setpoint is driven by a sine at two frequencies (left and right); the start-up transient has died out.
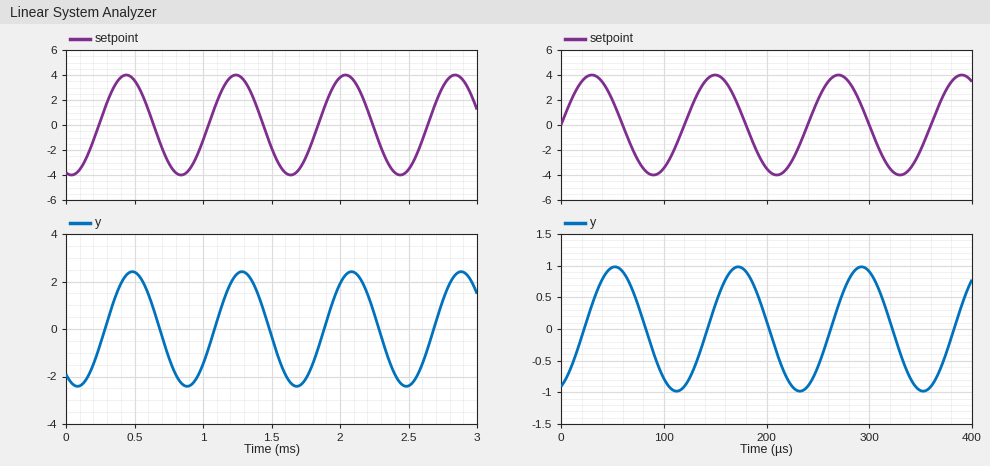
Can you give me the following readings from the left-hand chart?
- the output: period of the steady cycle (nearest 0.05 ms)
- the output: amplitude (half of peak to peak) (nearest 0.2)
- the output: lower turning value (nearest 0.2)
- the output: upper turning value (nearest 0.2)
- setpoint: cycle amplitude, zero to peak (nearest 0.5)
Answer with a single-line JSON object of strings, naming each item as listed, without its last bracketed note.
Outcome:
{"the output: period of the steady cycle": "0.80 ms", "the output: amplitude (half of peak to peak)": "2.4", "the output: lower turning value": "-2.4", "the output: upper turning value": "2.4", "setpoint: cycle amplitude, zero to peak": "4.0"}
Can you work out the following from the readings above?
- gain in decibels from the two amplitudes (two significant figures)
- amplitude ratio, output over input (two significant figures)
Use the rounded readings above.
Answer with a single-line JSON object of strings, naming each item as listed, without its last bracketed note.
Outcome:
{"gain in decibels from the two amplitudes": "-4.4 dB", "amplitude ratio, output over input": "0.60"}
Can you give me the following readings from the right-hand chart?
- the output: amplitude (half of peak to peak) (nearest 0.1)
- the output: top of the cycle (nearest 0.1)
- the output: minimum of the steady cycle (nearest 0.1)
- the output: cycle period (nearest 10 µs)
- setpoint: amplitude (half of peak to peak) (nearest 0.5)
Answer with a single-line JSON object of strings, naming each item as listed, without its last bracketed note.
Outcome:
{"the output: amplitude (half of peak to peak)": "1.0", "the output: top of the cycle": "1.0", "the output: minimum of the steady cycle": "-1.0", "the output: cycle period": "120 µs", "setpoint: amplitude (half of peak to peak)": "4.0"}
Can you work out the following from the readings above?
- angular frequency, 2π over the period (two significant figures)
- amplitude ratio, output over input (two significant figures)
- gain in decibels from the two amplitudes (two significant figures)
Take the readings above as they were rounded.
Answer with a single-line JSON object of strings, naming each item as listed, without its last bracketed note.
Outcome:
{"angular frequency, 2π over the period": "0.052 rad/µs", "amplitude ratio, output over input": "0.25", "gain in decibels from the two amplitudes": "-12 dB"}
